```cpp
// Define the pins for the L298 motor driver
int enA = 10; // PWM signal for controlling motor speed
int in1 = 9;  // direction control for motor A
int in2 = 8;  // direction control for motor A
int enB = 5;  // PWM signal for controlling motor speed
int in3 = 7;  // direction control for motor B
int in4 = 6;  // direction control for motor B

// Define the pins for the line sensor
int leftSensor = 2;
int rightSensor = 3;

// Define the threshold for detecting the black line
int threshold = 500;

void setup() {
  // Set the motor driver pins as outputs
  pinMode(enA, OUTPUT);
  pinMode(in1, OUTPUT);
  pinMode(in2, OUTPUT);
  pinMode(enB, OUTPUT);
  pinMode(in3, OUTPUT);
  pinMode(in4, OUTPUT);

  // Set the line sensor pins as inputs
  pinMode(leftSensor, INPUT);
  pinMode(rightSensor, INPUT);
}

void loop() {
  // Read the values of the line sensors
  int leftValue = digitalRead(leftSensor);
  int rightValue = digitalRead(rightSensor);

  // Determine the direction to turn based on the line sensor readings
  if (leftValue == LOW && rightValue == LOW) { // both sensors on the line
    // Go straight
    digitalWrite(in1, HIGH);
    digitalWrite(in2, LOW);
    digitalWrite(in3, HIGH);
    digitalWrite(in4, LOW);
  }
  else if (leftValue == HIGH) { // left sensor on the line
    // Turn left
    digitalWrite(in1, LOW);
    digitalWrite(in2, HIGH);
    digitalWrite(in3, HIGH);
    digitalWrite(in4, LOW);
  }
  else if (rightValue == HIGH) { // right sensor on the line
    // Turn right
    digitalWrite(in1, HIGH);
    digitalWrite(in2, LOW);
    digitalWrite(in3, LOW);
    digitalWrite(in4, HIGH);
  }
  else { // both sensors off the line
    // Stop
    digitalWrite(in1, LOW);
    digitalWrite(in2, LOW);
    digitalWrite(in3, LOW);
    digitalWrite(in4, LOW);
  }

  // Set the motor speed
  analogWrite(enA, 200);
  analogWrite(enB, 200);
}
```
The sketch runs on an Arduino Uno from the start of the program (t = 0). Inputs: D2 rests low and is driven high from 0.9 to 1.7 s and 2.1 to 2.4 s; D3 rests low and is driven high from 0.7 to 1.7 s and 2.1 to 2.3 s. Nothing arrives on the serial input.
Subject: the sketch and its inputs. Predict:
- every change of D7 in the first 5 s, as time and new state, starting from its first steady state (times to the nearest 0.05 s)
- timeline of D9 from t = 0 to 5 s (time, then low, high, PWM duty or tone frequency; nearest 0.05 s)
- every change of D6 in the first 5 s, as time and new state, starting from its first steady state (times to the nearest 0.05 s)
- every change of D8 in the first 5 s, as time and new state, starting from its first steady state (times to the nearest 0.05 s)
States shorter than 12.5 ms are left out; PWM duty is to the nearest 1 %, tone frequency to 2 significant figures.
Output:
0 s high; 0.7 s low; 0.9 s high
0 s high; 0.9 s low; 1.7 s high; 2.1 s low; 2.4 s high
0 s low; 0.7 s high; 0.9 s low
0 s low; 0.9 s high; 1.7 s low; 2.1 s high; 2.4 s low
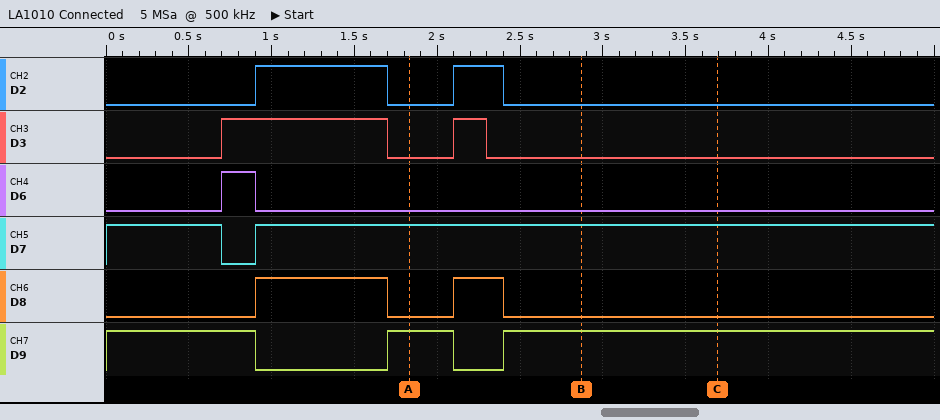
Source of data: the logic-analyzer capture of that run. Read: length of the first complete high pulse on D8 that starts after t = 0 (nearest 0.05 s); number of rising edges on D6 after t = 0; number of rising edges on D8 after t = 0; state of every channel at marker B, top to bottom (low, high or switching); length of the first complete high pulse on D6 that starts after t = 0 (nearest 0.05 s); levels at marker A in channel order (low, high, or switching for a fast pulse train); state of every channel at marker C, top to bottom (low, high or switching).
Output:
0.80 s
1
2
D2 low, D3 low, D6 low, D7 high, D8 low, D9 high
0.20 s
D2 low, D3 low, D6 low, D7 high, D8 low, D9 high
D2 low, D3 low, D6 low, D7 high, D8 low, D9 high
